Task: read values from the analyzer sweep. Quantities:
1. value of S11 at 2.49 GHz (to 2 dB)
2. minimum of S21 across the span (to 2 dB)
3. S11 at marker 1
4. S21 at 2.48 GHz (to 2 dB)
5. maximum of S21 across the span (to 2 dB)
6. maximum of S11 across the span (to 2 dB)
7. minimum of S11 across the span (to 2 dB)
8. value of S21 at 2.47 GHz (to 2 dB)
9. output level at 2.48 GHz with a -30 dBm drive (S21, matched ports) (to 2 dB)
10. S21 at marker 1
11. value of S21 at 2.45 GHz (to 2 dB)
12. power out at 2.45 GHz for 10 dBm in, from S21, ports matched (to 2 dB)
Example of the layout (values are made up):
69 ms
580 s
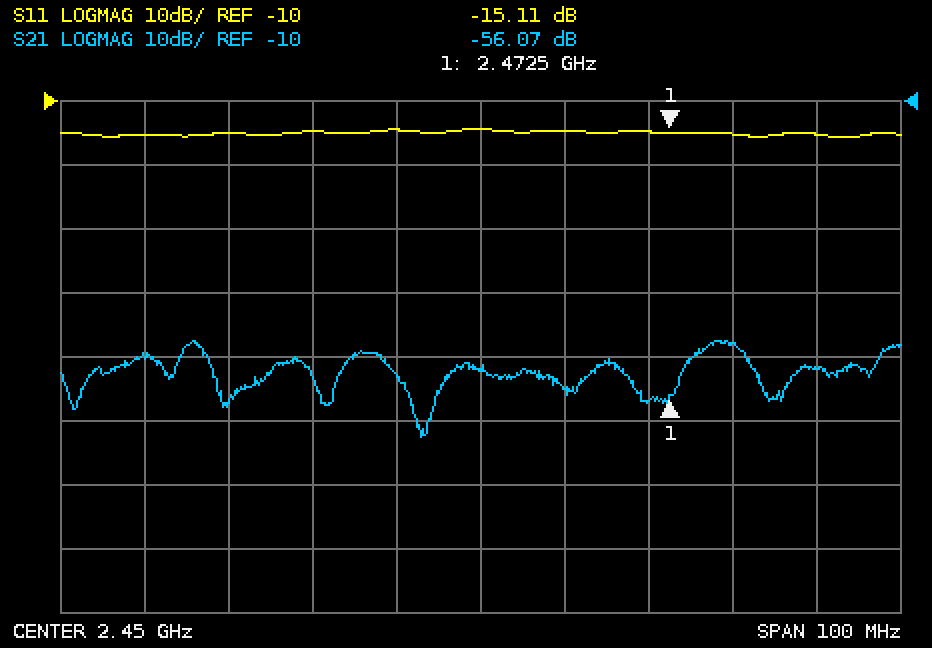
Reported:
-16 dB
-62 dB
-15.11 dB
-48 dB
-48 dB
-14 dB
-16 dB
-56 dB
-78 dBm
-56.07 dB
-52 dB
-42 dBm
